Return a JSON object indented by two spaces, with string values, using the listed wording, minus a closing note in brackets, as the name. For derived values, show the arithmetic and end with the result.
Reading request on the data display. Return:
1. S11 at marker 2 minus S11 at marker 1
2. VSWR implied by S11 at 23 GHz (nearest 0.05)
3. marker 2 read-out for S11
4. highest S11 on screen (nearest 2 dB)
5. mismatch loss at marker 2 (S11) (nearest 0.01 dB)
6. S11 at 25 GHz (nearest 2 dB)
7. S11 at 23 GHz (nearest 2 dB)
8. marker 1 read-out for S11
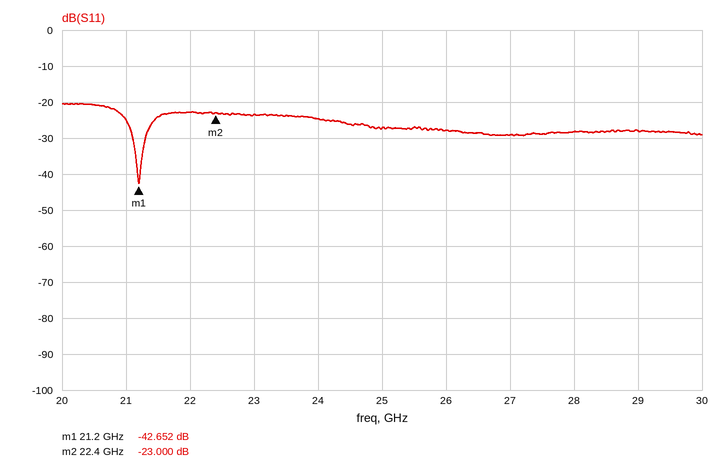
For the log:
{
  "S11 at marker 2 minus S11 at marker 1": "-23 − (-42.652) = 19.652 dB",
  "VSWR implied by S11 at 23 GHz": "|Γ| = 10^(-24/20) = 0.0631; VSWR = (1 + 0.0631)/(1 − 0.0631) ≈ 1.13, so 1.15 to the nearest 0.05",
  "marker 2 read-out for S11": "-23.000 dB",
  "highest S11 on screen": "-20 dB",
  "mismatch loss at marker 2 (S11)": "−10 log10(1 − 10^(-23/10)) ≈ 0.02 dB",
  "S11 at 25 GHz": "-28 dB",
  "S11 at 23 GHz": "-24 dB",
  "marker 1 read-out for S11": "-42.652 dB"
}
